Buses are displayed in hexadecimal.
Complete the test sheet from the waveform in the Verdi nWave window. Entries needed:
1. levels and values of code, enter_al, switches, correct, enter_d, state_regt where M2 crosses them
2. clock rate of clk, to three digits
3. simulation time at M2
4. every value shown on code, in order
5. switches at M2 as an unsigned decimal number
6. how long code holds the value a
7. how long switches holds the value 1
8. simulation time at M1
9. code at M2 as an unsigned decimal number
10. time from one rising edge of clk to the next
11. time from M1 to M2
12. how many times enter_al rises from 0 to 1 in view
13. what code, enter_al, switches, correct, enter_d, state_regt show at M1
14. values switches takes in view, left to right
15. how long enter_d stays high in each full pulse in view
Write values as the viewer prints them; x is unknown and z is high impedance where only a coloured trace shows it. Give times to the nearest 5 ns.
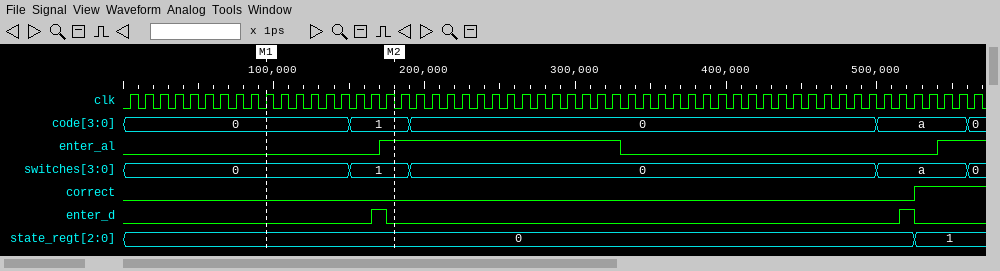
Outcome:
code=1, enter_al=1, switches=1, correct=0, enter_d=0, state_regt=0
100 MHz
180 ns
0, 1, 0, a, 0
1
60 ns
40 ns
95 ns
1
10 ns
85 ns
2
code=0, enter_al=0, switches=0, correct=0, enter_d=0, state_regt=0
0, 1, 0, a, 0
10 ns, 10 ns
